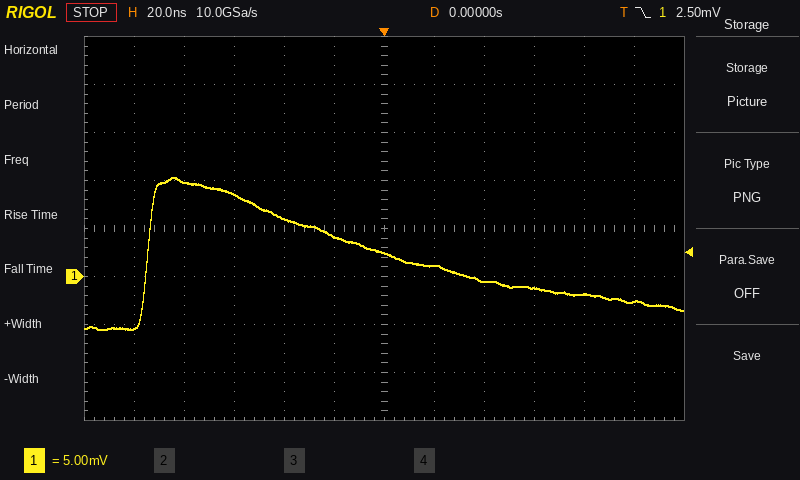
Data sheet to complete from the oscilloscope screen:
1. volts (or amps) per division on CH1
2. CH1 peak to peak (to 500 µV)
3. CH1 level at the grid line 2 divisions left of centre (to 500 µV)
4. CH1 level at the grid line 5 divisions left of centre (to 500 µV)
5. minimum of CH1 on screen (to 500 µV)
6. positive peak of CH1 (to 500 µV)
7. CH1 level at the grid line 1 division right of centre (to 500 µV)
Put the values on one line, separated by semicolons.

5 mV; 16.0 mV; 6.0 mV; -5.5 mV; -5.5 mV; 10.5 mV; 1.0 mV
